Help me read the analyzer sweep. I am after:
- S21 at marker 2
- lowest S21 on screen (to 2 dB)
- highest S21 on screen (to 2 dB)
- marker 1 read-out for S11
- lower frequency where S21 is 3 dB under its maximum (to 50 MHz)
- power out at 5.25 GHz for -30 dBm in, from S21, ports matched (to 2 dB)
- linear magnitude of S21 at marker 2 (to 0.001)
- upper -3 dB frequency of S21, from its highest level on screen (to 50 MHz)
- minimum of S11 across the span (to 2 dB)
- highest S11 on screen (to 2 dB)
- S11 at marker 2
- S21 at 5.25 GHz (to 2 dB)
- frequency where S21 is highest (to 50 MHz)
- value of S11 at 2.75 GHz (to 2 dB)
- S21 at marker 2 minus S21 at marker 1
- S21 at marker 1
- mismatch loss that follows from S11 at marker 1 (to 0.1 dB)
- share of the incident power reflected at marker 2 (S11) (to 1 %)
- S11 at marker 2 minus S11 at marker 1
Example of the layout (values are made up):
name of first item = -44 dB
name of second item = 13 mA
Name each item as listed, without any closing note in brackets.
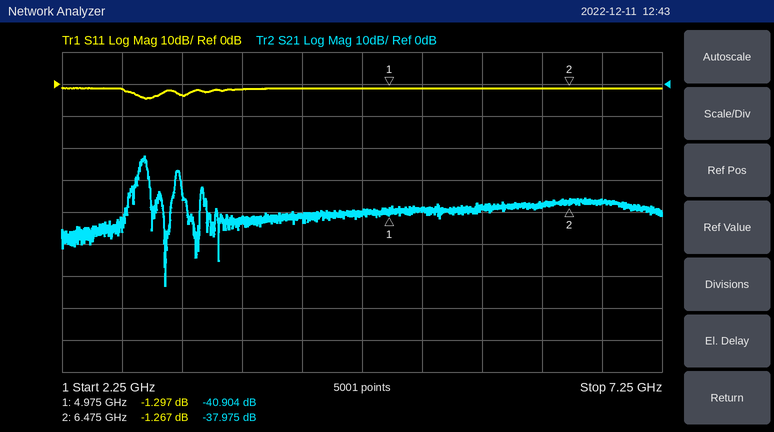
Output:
S21 at marker 2 = -37.975 dB
lowest S21 on screen = -64 dB
highest S21 on screen = -22 dB
marker 1 read-out for S11 = -1.297 dB
lower frequency where S21 is 3 dB under its maximum = 2.90 GHz
power out at 5.25 GHz for -30 dBm in, from S21, ports matched = -70 dBm
linear magnitude of S21 at marker 2 = 0.013
upper -3 dB frequency of S21, from its highest level on screen = 2.95 GHz
minimum of S11 across the span = -4 dB
highest S11 on screen = -2 dB
S11 at marker 2 = -1.267 dB
S21 at 5.25 GHz = -40 dB
frequency where S21 is highest = 2.95 GHz
value of S11 at 2.75 GHz = -2 dB
S21 at marker 2 minus S21 at marker 1 = 2.929 dB
S21 at marker 1 = -40.904 dB
mismatch loss that follows from S11 at marker 1 = 5.9 dB
share of the incident power reflected at marker 2 (S11) = 75 %
S11 at marker 2 minus S11 at marker 1 = 0.030 dB
